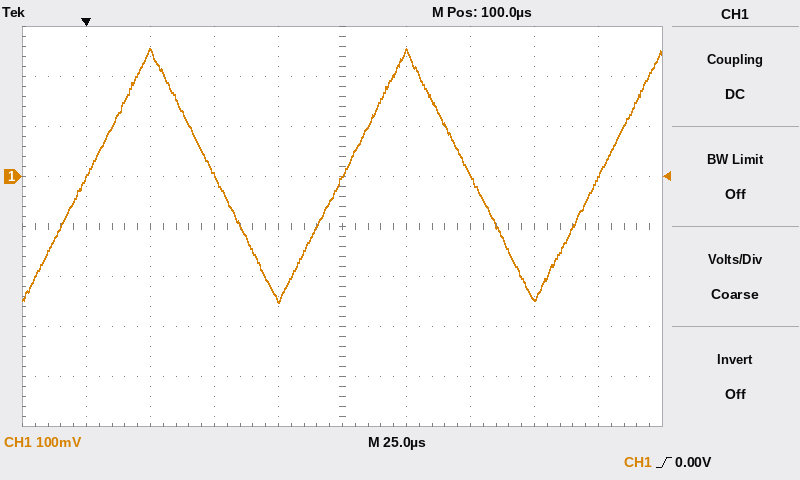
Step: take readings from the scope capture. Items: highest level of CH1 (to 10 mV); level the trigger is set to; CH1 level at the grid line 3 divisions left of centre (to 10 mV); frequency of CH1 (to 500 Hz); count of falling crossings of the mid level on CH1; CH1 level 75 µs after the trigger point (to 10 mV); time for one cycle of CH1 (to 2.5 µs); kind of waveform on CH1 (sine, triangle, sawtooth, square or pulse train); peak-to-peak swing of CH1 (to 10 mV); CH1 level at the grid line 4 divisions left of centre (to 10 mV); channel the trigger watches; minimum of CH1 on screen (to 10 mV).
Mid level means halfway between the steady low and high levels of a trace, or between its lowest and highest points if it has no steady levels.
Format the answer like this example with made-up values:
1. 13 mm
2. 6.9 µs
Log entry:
1. 260 mV
2. 0.00 V
3. 250 mV
4. 10.0 kHz
5. 2
6. -240 mV
7. 100.0 µs
8. triangle
9. 510 mV
10. 0 mV
11. CH1
12. -250 mV
